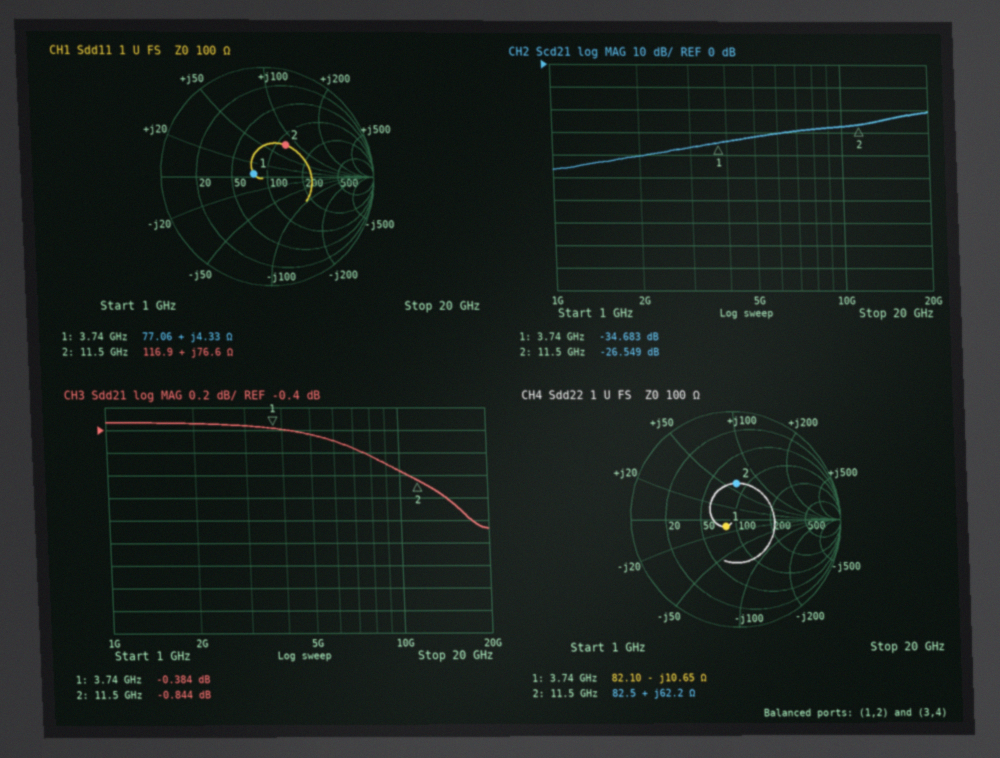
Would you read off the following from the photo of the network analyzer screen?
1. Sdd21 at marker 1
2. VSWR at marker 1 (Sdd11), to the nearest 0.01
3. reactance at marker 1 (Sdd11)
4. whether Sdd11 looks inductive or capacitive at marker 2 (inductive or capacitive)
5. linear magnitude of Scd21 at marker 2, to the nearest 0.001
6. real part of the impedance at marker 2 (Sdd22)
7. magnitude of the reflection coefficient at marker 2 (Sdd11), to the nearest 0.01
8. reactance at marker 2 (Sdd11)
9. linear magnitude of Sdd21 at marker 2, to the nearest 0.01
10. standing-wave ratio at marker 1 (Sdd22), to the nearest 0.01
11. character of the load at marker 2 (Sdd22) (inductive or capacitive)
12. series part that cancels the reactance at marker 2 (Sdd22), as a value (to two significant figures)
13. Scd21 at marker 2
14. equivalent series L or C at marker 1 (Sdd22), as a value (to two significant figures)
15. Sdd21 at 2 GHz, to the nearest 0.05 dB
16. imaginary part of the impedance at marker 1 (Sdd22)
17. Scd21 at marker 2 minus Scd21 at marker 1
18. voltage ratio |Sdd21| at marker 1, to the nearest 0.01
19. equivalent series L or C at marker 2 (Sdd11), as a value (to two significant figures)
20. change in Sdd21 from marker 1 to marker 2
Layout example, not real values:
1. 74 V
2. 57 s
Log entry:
1. -0.384 dB
2. 1.30
3. +4.33 Ω
4. inductive
5. 0.047
6. 82.5 Ω
7. 0.34
8. +76.6 Ω
9. 0.91
10. 1.26
11. inductive
12. 220 fF
13. -26.549 dB
14. 4.0 pF
15. -0.35 dB
16. -10.65 Ω
17. 8.134 dB
18. 0.96
19. 1.1 nH
20. -0.460 dB
